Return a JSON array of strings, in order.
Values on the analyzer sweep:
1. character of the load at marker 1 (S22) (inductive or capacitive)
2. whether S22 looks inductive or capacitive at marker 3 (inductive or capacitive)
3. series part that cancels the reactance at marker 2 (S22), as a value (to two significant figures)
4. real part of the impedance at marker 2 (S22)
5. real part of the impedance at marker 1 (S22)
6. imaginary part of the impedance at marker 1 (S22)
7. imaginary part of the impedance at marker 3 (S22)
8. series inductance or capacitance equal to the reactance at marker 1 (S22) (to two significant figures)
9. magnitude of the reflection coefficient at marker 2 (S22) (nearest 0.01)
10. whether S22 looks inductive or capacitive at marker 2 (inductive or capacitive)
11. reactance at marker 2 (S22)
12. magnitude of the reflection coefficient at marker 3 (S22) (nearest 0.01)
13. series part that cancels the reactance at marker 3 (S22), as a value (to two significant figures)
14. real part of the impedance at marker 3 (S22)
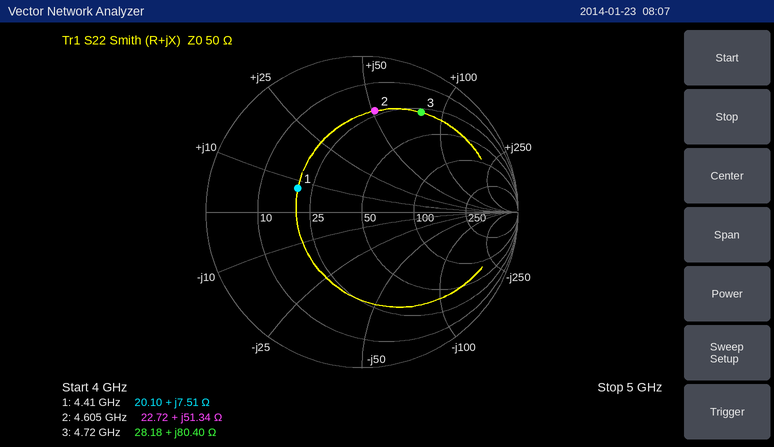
["inductive", "inductive", "670 fF", "22.72 Ω", "20.10 Ω", "+7.51 Ω", "+80.40 Ω", "270 pH", "0.65", "inductive", "+51.34 Ω", "0.74", "420 fF", "28.18 Ω"]
